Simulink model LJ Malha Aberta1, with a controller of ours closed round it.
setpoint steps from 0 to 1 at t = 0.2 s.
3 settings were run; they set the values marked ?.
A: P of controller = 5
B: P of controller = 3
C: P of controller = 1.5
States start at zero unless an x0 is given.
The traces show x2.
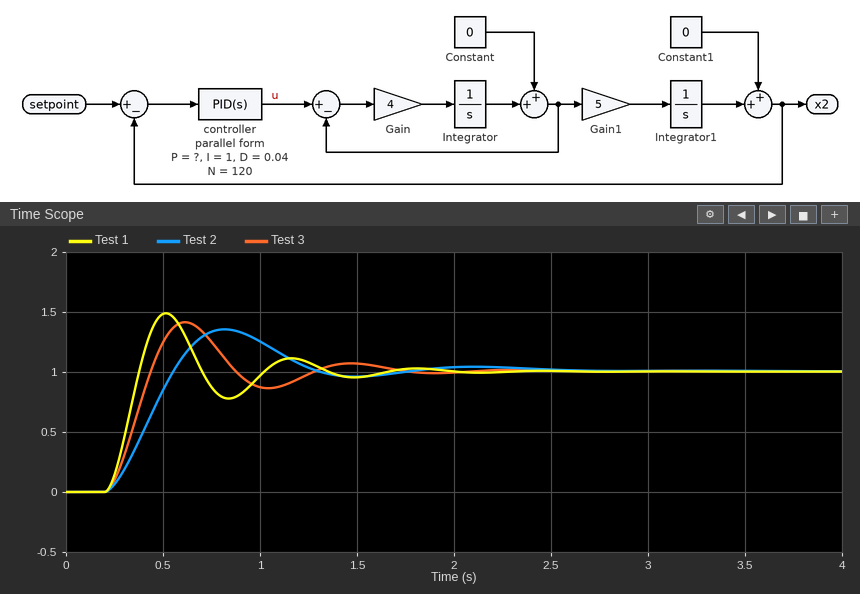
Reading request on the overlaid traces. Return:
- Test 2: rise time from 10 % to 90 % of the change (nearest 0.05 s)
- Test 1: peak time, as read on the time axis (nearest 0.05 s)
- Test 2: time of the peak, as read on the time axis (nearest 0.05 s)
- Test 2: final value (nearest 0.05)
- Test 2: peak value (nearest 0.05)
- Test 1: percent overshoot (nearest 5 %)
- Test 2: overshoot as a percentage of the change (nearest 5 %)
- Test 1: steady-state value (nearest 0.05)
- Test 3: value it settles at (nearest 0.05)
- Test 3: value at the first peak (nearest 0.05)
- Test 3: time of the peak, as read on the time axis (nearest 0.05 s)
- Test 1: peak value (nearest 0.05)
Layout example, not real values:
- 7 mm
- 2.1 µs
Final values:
- 0.25 s
- 0.50 s
- 0.80 s
- 1.00
- 1.35
- 50 %
- 35 %
- 1.00
- 1.00
- 1.40
- 0.60 s
- 1.50
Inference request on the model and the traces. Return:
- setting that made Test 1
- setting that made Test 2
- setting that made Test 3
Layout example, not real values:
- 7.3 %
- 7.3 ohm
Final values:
- A
- C
- B
